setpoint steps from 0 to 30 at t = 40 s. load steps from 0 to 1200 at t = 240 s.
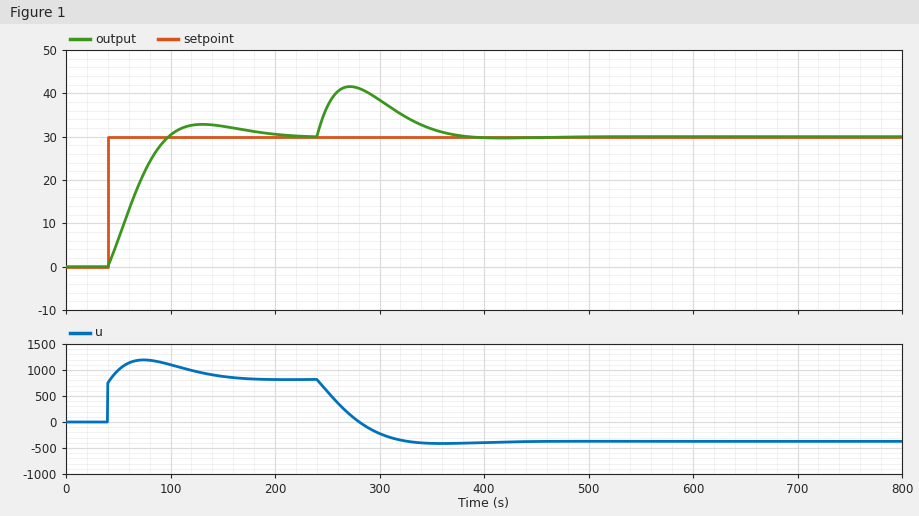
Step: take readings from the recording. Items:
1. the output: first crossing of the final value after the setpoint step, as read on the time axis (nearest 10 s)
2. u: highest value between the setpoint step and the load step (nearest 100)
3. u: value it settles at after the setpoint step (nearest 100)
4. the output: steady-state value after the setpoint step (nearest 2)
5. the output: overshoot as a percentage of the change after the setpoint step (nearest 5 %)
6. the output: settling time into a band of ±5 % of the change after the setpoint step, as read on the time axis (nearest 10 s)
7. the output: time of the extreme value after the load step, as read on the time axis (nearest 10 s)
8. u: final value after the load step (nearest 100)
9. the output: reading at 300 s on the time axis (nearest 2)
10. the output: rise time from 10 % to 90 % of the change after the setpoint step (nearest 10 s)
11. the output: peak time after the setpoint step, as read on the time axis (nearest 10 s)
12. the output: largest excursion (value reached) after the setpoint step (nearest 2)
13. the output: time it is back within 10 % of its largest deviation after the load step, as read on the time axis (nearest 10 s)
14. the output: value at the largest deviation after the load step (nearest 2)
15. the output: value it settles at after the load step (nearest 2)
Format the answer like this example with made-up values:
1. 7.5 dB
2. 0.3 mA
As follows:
1. 100 s
2. 1200
3. 800
4. 30
5. 10 %
6. 170 s
7. 270 s
8. -400
9. 38
10. 40 s
11. 130 s
12. 32
13. 360 s
14. 42
15. 30
